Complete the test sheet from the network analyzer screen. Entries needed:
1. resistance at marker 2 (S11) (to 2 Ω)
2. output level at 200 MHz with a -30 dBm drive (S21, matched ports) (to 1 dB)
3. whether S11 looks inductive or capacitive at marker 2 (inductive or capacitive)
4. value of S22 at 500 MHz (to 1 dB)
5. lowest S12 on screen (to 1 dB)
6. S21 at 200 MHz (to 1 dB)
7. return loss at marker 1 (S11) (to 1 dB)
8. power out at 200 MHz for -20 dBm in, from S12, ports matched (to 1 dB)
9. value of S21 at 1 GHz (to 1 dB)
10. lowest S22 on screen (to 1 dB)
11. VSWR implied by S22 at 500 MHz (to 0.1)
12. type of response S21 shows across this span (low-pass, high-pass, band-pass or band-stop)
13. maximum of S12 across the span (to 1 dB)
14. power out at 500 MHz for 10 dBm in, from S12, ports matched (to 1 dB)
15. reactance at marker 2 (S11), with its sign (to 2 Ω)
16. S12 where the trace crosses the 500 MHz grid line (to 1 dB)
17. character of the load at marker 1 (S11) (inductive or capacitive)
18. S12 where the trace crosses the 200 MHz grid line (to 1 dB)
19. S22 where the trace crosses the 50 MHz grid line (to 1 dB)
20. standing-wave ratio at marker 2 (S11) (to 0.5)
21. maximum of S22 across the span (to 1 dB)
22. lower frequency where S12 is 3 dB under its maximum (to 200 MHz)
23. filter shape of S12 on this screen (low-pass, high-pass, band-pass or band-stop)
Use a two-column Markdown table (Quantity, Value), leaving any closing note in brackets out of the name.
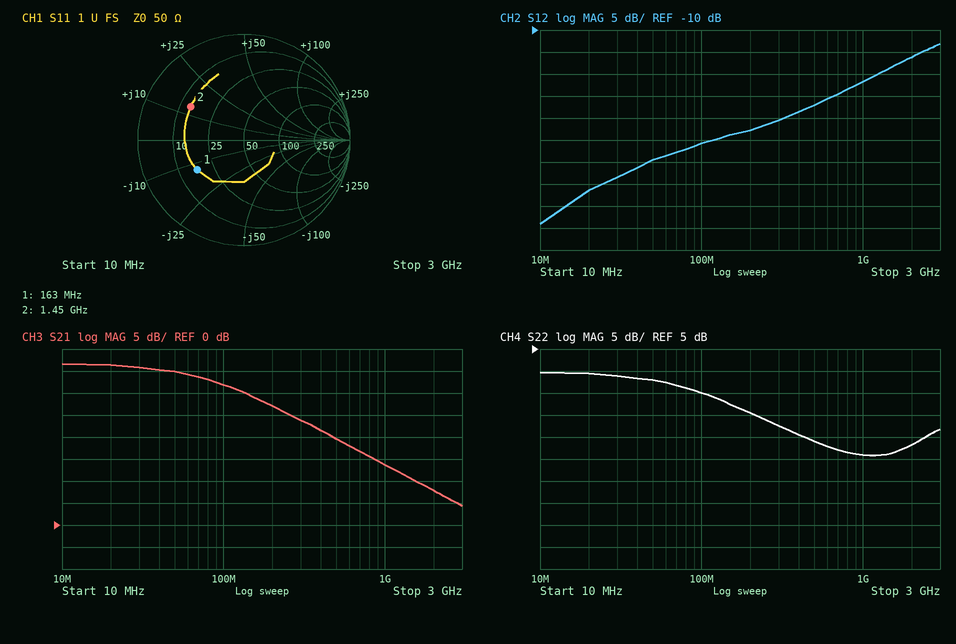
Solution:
| Quantity | Value |
|---|---|
| resistance at marker 2 (S11) | 14 Ω |
| output level at 200 MHz with a -30 dBm drive (S21, matched ports) | -3 dBm |
| whether S11 looks inductive or capacitive at marker 2 | inductive |
| value of S22 at 500 MHz | -16 dB |
| lowest S12 on screen | -54 dB |
| S21 at 200 MHz | 27 dB |
| return loss at marker 1 (S11) | 6 dB |
| power out at 200 MHz for -20 dBm in, from S12, ports matched | -53 dBm |
| value of S21 at 1 GHz | 14 dB |
| lowest S22 on screen | -19 dB |
| VSWR implied by S22 at 500 MHz | 1.4 |
| type of response S21 shows across this span | low-pass |
| maximum of S12 across the span | -13 dB |
| power out at 500 MHz for 10 dBm in, from S12, ports matched | -17 dBm |
| reactance at marker 2 (S11), with its sign | +14 Ω |
| S12 where the trace crosses the 500 MHz grid line | -27 dB |
| character of the load at marker 1 (S11) | capacitive |
| S12 where the trace crosses the 200 MHz grid line | -33 dB |
| S22 where the trace crosses the 50 MHz grid line | -2 dB |
| standing-wave ratio at marker 2 (S11) | 4.0 |
| maximum of S22 across the span | 0 dB |
| lower frequency where S12 is 3 dB under its maximum | 2.0 GHz |
| filter shape of S12 on this screen | high-pass |
